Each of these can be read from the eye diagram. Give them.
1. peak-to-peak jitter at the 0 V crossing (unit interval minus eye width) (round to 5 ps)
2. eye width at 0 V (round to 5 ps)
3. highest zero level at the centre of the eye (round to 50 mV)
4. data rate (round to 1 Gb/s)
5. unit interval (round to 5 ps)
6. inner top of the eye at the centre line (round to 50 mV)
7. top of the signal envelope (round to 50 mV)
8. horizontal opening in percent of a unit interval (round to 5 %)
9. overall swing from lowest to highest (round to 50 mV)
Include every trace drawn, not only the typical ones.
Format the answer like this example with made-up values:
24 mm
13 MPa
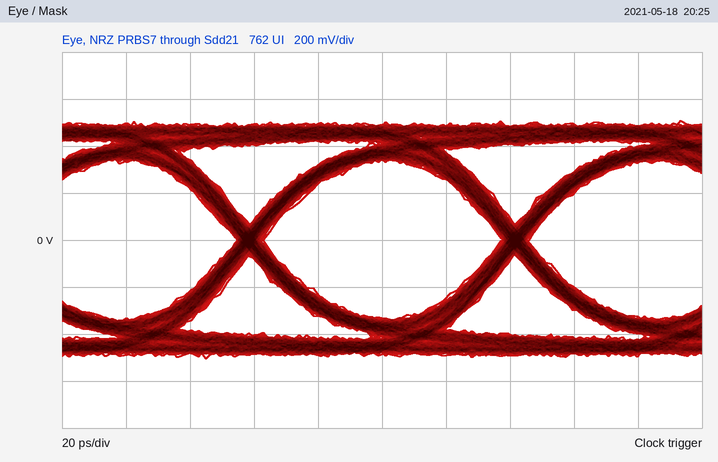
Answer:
10 ps
75 ps
-350 mV
12 Gb/s
85 ps
350 mV
500 mV
90 %
1.00 V
